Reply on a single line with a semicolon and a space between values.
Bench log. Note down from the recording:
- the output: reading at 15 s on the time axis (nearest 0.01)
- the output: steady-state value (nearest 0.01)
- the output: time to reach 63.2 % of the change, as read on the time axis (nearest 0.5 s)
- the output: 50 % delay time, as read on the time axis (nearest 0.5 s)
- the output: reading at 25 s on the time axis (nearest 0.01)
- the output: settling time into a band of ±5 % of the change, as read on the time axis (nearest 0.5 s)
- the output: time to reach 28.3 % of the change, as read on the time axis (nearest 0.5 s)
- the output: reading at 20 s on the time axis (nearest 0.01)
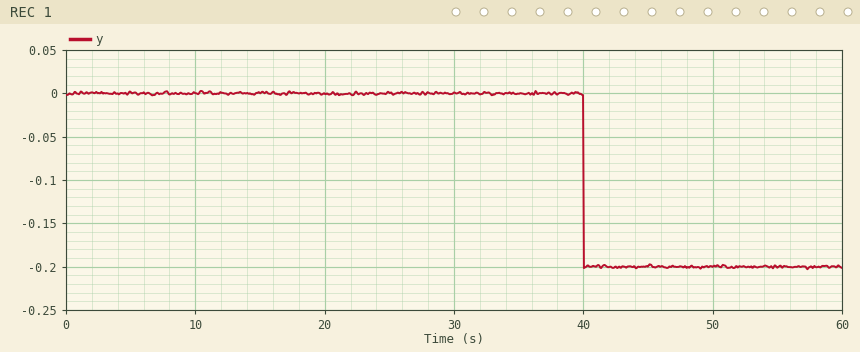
0.00; -0.20; 40.0 s; 40.0 s; 0.00; 40.0 s; 40.0 s; 0.00
